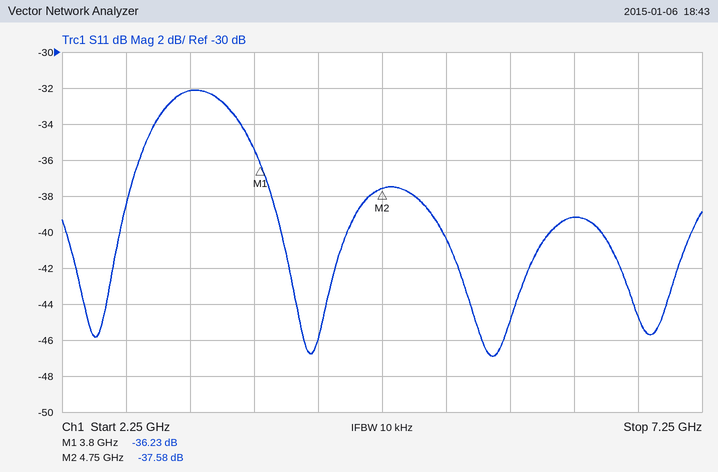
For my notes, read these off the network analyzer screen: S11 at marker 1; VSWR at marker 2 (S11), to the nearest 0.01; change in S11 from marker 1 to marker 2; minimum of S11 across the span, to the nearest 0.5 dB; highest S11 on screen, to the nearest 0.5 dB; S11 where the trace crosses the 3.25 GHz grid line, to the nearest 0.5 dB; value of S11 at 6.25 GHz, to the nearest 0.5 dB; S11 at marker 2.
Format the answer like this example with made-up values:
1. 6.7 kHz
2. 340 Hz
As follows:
1. -36.23 dB
2. 1.03
3. -1.35 dB
4. -47.0 dB
5. -32.0 dB
6. -32.0 dB
7. -39.0 dB
8. -37.58 dB
